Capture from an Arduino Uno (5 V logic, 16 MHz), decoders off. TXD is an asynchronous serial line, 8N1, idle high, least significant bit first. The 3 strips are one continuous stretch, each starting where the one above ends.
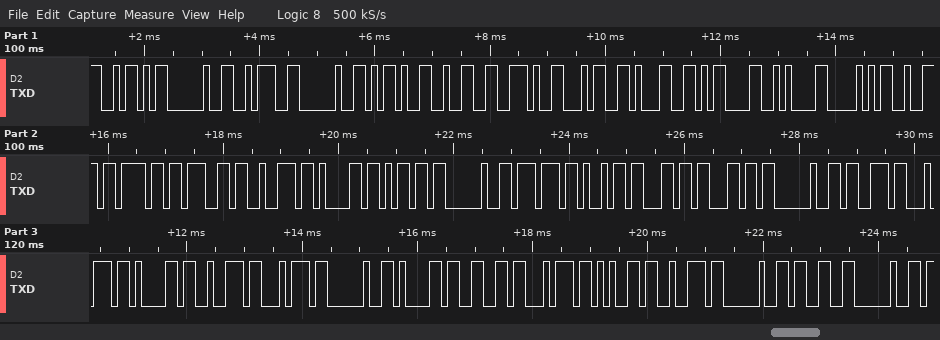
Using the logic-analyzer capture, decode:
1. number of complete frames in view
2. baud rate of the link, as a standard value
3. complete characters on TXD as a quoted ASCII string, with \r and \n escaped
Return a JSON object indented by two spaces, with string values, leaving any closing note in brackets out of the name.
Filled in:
{
  "number of complete frames in view": "38",
  "baud rate of the link, as a standard value": "9600 baud",
  "complete characters on TXD as a quoted ASCII string, with \\r and \\n escaped": "\"Z : -2.41\\r\\nProgram will start after 3 \""
}
